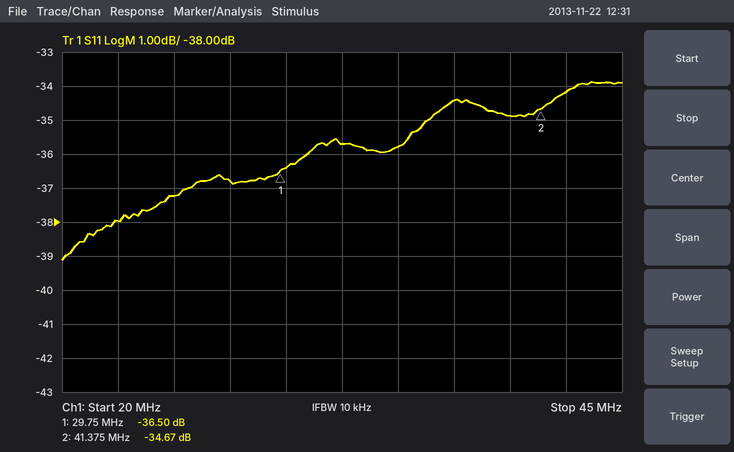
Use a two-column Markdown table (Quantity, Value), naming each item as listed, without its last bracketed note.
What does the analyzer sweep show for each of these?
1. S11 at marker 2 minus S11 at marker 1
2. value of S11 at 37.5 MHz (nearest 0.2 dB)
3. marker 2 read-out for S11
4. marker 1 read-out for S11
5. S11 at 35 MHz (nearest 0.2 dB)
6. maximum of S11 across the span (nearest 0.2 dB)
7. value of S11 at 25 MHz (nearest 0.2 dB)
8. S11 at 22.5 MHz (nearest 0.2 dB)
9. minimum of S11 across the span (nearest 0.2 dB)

| Quantity | Value |
|---|---|
| S11 at marker 2 minus S11 at marker 1 | 1.83 dB |
| value of S11 at 37.5 MHz | -34.4 dB |
| marker 2 read-out for S11 | -34.67 dB |
| marker 1 read-out for S11 | -36.50 dB |
| S11 at 35 MHz | -35.8 dB |
| maximum of S11 across the span | -33.8 dB |
| value of S11 at 25 MHz | -37.2 dB |
| S11 at 22.5 MHz | -38.0 dB |
| minimum of S11 across the span | -39.2 dB |
